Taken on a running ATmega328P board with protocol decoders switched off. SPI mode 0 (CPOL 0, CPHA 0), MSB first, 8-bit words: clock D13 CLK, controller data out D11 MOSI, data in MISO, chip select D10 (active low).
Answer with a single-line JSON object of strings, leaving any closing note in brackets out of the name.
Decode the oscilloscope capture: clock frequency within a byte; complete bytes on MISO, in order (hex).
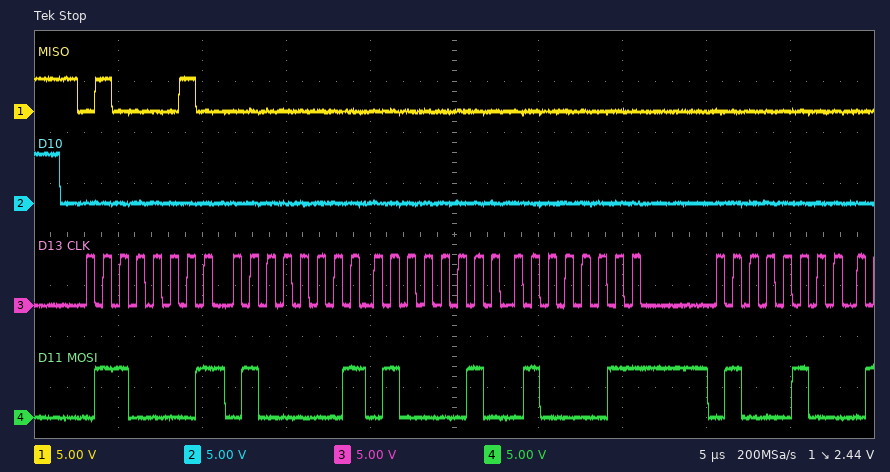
{"clock frequency within a byte": "1 MHz", "complete bytes on MISO, in order": "42 00 00 00 00"}
